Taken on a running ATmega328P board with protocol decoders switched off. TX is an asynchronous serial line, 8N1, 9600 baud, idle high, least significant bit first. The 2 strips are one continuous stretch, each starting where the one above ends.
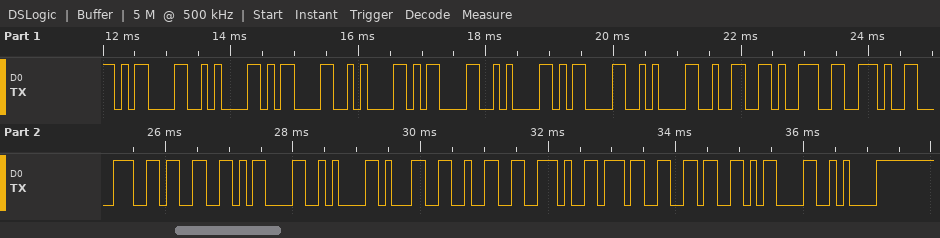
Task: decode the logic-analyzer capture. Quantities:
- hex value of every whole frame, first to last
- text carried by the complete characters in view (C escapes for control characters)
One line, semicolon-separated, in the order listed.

0D 0A 0D 0A 0D 0A 0D 0A 32 39 2E 38 33 0D 0A 31 32 2E 37 36 0D 0A; "\r\n\r\n\r\n\r\n29.83\r\n12.76\r\n"
